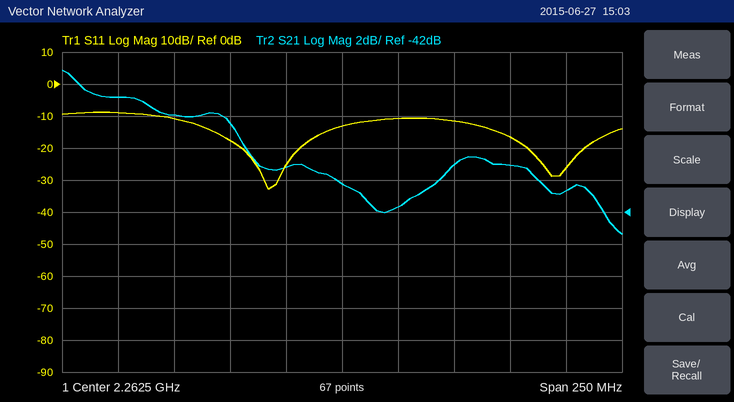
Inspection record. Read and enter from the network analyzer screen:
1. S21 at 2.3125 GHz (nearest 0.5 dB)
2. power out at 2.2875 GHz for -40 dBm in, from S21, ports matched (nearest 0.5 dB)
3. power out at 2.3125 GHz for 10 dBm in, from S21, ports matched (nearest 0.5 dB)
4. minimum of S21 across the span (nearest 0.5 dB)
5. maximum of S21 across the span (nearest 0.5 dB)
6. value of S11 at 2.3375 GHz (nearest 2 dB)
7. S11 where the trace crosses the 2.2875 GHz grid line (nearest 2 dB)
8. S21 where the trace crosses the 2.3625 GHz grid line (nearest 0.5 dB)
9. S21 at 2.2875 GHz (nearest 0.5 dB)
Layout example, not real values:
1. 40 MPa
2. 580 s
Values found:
1. -39.0 dB
2. -81.5 dBm
3. -29.0 dBm
4. -43.5 dB
5. -33.0 dB
6. -16 dB
7. -10 dB
8. -40.5 dB
9. -41.5 dB
